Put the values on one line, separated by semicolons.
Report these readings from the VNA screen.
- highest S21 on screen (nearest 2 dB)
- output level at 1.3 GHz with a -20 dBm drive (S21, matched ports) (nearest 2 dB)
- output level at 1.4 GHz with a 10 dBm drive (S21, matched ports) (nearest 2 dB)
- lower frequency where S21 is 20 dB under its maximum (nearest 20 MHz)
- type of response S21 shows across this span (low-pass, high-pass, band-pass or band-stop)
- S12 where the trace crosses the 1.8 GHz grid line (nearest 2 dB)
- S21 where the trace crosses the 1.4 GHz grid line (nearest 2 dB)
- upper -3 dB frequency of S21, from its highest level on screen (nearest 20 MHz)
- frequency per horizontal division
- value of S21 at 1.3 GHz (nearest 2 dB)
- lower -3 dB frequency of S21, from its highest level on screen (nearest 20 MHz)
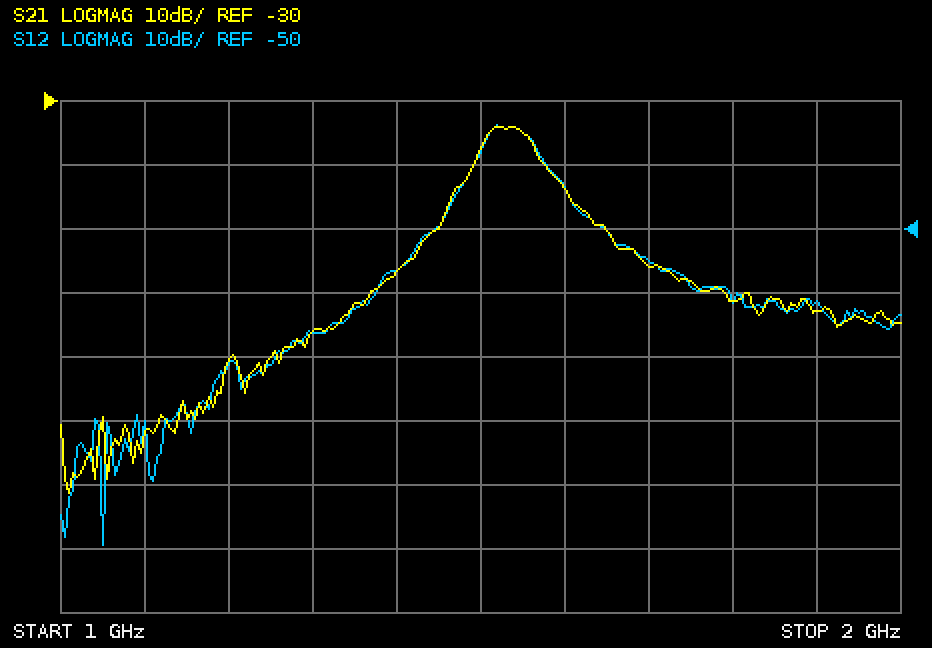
-34 dB; -86 dBm; -46 dBm; 1.42 GHz; band-pass; -62 dB; -56 dB; 1.56 GHz; 100 MHz; -66 dB; 1.50 GHz
